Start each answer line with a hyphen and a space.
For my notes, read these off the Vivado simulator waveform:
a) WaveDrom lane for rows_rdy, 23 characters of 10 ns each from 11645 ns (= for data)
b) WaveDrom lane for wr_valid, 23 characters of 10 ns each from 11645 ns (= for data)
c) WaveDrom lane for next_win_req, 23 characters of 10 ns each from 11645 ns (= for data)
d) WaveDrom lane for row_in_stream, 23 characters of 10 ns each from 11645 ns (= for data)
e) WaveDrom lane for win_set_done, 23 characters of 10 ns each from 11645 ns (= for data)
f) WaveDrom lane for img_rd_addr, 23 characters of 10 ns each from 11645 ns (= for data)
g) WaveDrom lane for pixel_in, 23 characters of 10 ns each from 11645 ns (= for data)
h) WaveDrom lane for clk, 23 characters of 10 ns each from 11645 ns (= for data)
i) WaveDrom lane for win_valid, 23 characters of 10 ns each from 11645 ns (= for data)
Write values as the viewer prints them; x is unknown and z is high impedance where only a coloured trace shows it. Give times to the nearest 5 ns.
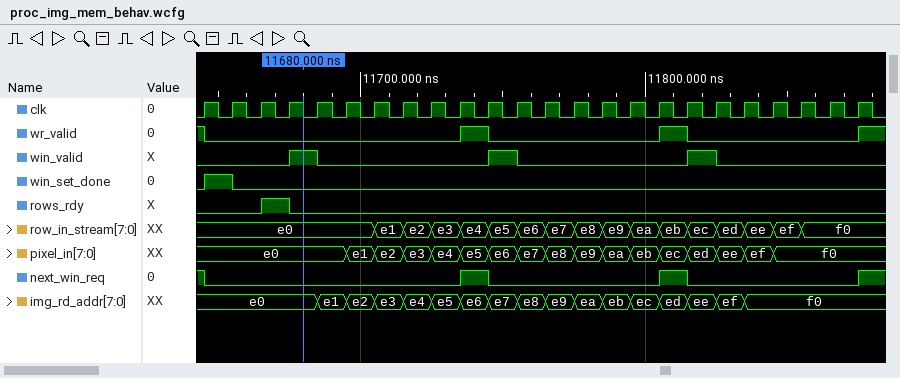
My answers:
- {name: 'rows_rdy', wave: '0.10...................'}
- {name: 'wr_valid', wave: '0........10.....10.....'}
- {name: 'next_win_req', wave: '0........10.....10.....'}
- {name: 'row_in_stream', wave: '=.....================.', data: 'e0 e1 e2 e3 e4 e5 e6 e7 e8 e9 ea eb ec ed ee ef f0'}
- {name: 'win_set_done', wave: '10.....................'}
- {name: 'img_rd_addr', wave: '=...================...', data: 'e0 e1 e2 e3 e4 e5 e6 e7 e8 e9 ea eb ec ed ee ef f0'}
- {name: 'pixel_in', wave: '=....================..', data: 'e0 e1 e2 e3 e4 e5 e6 e7 e8 e9 ea eb ec ed ee ef f0'}
- {name: 'clk', wave: 'p......................'}
- {name: 'win_valid', wave: '0..10.....10.....10....'}
